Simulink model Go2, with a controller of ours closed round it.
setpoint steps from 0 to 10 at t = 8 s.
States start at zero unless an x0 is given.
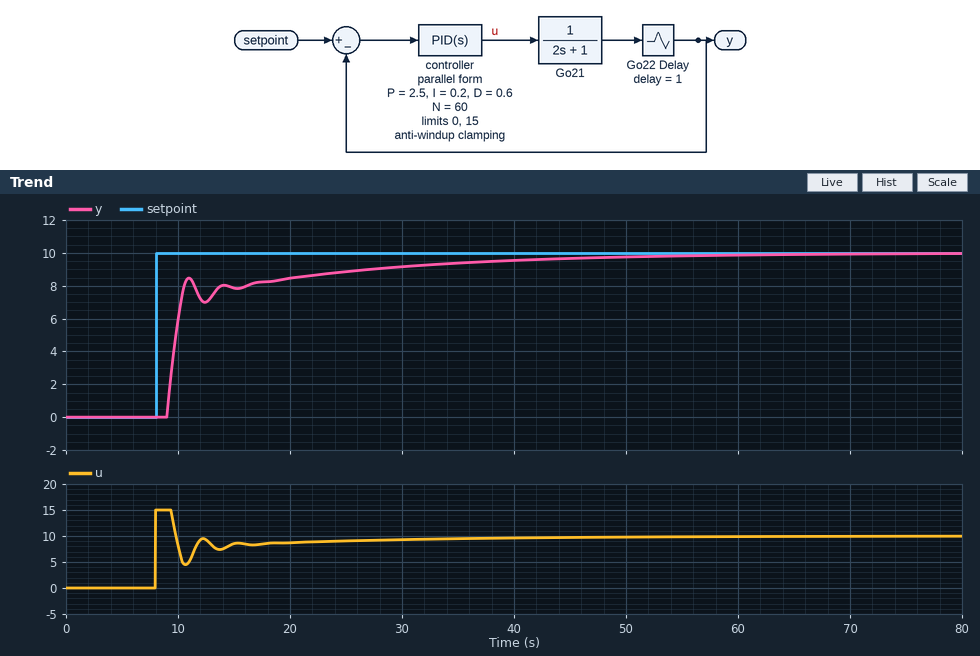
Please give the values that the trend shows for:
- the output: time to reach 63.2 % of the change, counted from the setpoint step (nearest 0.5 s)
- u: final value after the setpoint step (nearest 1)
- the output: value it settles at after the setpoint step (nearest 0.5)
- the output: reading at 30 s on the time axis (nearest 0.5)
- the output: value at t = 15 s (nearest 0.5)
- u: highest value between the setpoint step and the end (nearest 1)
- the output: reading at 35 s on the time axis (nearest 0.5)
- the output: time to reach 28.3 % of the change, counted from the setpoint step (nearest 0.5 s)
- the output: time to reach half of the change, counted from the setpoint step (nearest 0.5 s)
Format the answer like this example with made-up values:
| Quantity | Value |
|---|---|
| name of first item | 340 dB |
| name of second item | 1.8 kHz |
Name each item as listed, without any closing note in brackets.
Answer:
| Quantity | Value |
|---|---|
| the output: time to reach 63.2 % of the change, counted from the setpoint step | 2.0 s |
| u: final value after the setpoint step | 10 |
| the output: value it settles at after the setpoint step | 10.0 |
| the output: reading at 30 s on the time axis | 9.0 |
| the output: value at t = 15 s | 8.0 |
| u: highest value between the setpoint step and the end | 15 |
| the output: reading at 35 s on the time axis | 9.5 |
| the output: time to reach 28.3 % of the change, counted from the setpoint step | 1.5 s |
| the output: time to reach half of the change, counted from the setpoint step | 2.0 s |
